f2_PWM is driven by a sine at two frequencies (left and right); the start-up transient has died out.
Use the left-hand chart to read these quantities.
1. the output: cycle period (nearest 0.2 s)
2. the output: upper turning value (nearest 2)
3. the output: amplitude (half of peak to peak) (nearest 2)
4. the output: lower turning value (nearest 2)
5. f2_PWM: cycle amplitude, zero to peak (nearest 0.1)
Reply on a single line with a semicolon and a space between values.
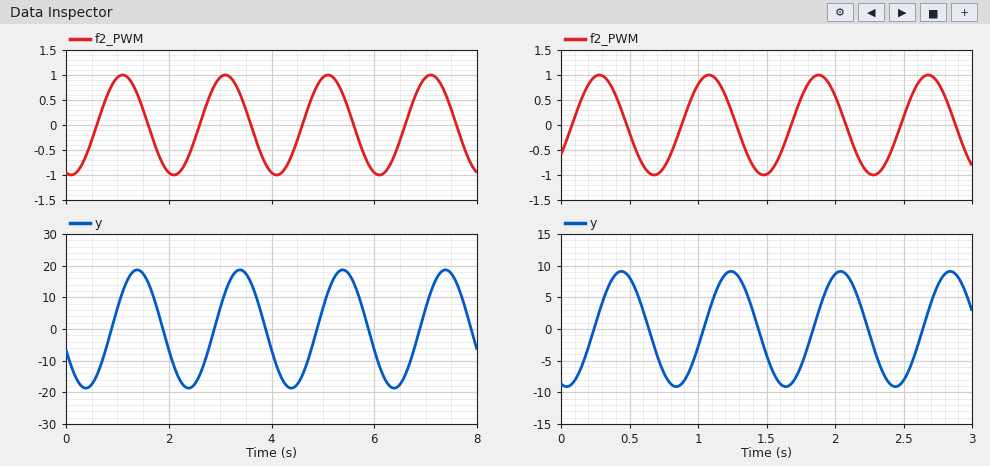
2.0 s; 18; 18; -18; 1.0
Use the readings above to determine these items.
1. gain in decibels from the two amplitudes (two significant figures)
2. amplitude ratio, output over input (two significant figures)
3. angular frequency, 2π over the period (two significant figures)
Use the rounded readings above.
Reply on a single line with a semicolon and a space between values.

25 dB; 18; 3.1 rad/s
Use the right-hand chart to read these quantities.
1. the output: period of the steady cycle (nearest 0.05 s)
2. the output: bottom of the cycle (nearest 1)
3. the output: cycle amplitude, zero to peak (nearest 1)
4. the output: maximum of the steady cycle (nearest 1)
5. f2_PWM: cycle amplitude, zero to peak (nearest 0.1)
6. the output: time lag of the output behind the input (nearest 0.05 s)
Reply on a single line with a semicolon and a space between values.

0.80 s; -9; 9; 9; 1.0; 0.15 s
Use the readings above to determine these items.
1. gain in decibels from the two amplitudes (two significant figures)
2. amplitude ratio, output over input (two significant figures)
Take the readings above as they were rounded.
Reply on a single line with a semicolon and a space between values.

19 dB; 9.0
